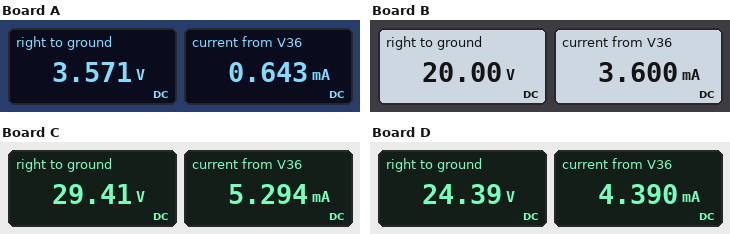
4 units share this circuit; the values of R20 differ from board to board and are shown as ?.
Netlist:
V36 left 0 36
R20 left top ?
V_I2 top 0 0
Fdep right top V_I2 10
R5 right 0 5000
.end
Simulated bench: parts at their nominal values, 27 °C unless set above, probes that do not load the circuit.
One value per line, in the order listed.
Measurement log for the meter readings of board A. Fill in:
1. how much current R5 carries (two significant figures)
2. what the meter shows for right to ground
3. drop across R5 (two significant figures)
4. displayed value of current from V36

710 µA
3.571 V
3.6 V
0.643 mA
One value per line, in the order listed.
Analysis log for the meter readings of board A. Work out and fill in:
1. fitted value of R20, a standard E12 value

56 kΩ
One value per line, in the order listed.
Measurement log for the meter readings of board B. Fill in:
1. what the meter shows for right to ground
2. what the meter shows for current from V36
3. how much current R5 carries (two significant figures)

20.00 V
3.600 mA
4.0 mA
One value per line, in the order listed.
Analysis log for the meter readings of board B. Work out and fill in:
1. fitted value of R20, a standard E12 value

10 kΩ
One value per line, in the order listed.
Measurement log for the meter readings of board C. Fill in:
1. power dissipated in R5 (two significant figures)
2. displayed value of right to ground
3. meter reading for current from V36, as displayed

170 mW
29.41 V
5.294 mA
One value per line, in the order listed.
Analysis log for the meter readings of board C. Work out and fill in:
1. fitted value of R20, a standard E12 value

6.8 kΩ
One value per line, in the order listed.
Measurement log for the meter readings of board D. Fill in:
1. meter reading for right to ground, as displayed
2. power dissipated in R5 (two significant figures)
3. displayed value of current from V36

24.39 V
120 mW
4.390 mA
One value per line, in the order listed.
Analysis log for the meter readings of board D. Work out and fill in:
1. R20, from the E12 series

8.2 kΩ
